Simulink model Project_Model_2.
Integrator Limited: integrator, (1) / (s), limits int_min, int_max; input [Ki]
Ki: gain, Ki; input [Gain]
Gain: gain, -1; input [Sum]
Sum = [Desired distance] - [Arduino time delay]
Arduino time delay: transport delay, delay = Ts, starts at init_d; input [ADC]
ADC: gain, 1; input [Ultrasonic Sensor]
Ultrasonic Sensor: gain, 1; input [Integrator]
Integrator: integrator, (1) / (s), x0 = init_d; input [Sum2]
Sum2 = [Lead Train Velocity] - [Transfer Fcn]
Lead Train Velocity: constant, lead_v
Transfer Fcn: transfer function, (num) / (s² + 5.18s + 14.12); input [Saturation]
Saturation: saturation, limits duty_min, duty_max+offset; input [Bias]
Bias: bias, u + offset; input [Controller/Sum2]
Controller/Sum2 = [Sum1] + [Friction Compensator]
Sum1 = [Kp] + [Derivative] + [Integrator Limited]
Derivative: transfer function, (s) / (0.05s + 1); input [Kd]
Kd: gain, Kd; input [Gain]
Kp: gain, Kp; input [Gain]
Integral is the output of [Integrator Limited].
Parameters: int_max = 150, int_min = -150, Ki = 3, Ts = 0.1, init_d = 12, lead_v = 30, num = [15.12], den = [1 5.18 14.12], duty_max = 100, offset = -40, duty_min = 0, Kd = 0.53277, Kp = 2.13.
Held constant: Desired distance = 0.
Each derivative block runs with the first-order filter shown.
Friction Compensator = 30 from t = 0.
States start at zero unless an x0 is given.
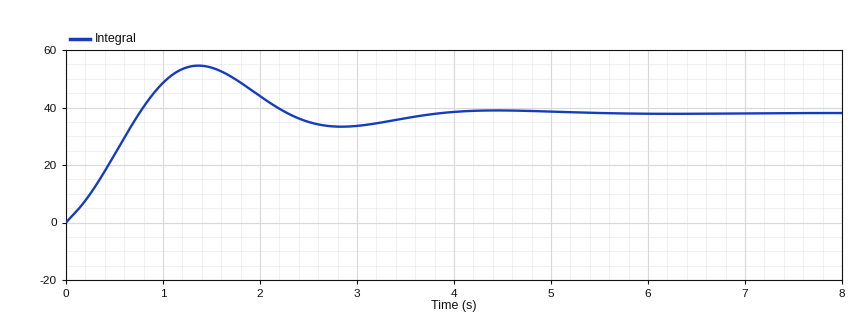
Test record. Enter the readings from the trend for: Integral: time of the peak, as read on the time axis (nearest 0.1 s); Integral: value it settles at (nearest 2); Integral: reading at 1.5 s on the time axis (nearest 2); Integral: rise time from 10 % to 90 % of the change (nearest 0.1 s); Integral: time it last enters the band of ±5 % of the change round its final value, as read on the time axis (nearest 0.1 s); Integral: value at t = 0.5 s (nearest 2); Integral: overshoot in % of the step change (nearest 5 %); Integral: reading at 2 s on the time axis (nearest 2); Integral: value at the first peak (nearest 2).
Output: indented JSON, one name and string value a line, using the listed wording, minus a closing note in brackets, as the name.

{
  "Integral: time of the peak, as read on the time axis": "1.4 s",
  "Integral: value it settles at": "38",
  "Integral: reading at 1.5 s on the time axis": "54",
  "Integral: rise time from 10 % to 90 % of the change": "0.6 s",
  "Integral: time it last enters the band of ±5 % of the change round its final value, as read on the time axis": "3.5 s",
  "Integral: value at t = 0.5 s": "24",
  "Integral: overshoot in % of the step change": "45 %",
  "Integral: reading at 2 s on the time axis": "44",
  "Integral: value at the first peak": "54"
}
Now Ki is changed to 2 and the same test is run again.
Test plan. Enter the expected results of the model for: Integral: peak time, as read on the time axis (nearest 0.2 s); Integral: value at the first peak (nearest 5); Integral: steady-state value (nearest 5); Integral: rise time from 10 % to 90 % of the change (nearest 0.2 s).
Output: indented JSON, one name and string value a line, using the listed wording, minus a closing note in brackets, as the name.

{
  "Integral: peak time, as read on the time axis": "1.8 s",
  "Integral: value at the first peak": "40",
  "Integral: steady-state value": "40",
  "Integral: rise time from 10 % to 90 % of the change": "0.8 s"
}
